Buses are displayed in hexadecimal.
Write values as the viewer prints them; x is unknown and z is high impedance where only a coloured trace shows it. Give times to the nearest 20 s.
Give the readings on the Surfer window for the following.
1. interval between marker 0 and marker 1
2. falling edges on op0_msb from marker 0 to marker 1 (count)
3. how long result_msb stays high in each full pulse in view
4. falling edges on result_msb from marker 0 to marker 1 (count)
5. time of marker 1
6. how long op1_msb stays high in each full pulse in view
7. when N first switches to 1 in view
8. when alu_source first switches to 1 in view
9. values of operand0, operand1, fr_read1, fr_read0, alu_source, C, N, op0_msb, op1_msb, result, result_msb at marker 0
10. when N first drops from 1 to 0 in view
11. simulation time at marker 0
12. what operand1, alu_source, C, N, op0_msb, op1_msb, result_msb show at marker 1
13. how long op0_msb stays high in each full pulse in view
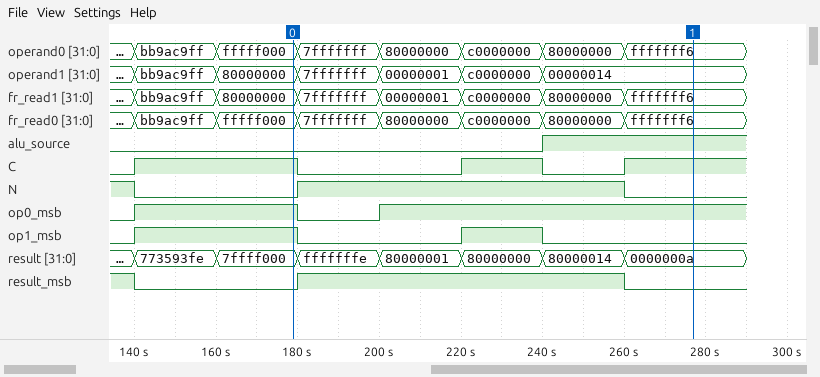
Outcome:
100 s
1
80 s
1
280 s
40 s, 20 s
180 s
240 s
operand0=fffff000, operand1=80000000, fr_read1=80000000, fr_read0=fffff000, alu_source=0, C=1, N=0, op0_msb=1, op1_msb=1, result=7ffff000, result_msb=0
140 s
180 s
operand1=00000014, alu_source=1, C=1, N=0, op0_msb=1, op1_msb=0, result_msb=0
40 s
